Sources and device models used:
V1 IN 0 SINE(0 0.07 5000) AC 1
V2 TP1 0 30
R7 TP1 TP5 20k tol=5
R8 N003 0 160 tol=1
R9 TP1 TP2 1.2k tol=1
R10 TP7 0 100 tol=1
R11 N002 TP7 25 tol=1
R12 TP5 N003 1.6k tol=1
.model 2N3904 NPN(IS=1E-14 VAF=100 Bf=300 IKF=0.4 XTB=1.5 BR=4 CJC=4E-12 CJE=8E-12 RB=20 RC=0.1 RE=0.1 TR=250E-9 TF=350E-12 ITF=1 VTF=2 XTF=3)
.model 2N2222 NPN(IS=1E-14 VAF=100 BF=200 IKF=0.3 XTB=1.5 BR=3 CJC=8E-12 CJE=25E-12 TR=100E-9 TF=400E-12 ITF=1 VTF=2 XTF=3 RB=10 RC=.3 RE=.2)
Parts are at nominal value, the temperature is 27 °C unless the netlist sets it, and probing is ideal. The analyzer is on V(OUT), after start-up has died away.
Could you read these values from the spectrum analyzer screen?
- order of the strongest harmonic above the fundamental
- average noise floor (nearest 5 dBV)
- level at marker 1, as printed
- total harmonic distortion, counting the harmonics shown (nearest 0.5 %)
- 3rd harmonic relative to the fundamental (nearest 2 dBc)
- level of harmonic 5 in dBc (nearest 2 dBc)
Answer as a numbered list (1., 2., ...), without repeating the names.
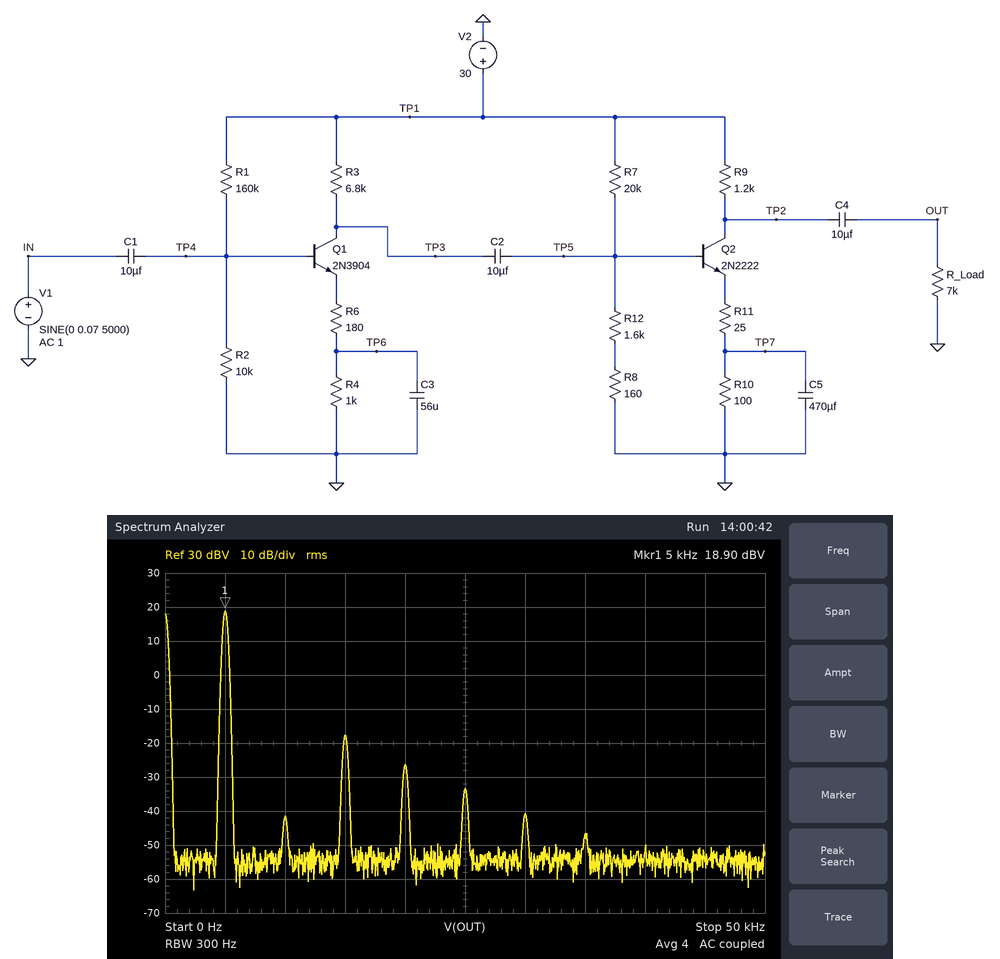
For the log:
1. 3
2. -55 dBV
3. 18.90 dBV
4. 1.5 %
5. -36 dBc
6. -52 dBc
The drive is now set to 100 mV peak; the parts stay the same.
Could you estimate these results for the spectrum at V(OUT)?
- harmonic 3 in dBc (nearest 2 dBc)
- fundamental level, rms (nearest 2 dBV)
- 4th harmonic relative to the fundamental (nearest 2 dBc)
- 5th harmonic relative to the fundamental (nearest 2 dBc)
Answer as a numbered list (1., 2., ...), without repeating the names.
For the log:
1. -18 dBc
2. 20 dBV
3. -56 dBc
4. -34 dBc
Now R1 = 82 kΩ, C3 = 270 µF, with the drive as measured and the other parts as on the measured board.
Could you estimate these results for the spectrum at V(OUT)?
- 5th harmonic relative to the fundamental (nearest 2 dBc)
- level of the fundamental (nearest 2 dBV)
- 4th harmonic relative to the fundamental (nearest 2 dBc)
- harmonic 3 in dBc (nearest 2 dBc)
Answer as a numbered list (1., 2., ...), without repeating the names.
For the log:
1. -38 dBc
2. 20 dBV
3. -58 dBc
4. -30 dBc
